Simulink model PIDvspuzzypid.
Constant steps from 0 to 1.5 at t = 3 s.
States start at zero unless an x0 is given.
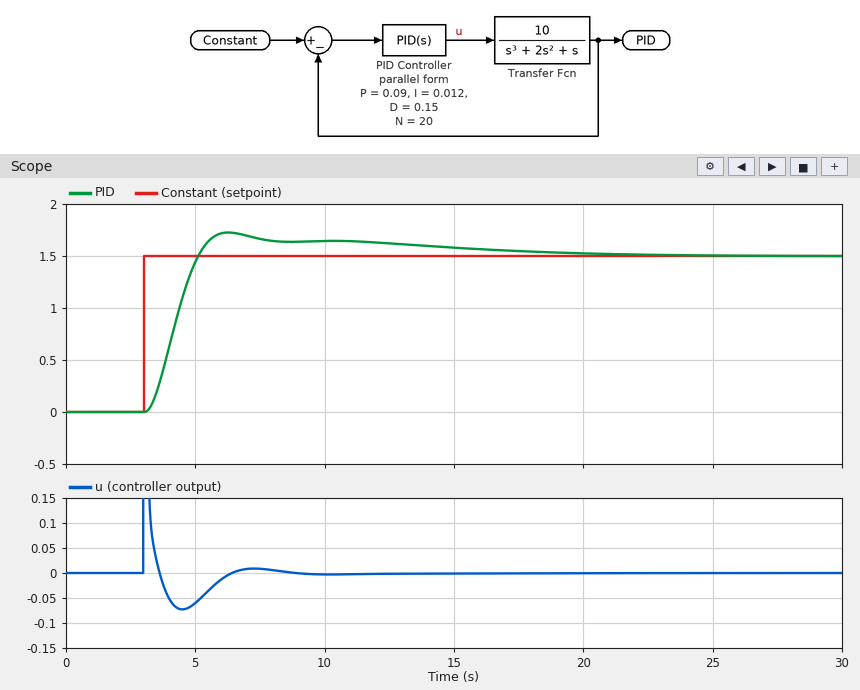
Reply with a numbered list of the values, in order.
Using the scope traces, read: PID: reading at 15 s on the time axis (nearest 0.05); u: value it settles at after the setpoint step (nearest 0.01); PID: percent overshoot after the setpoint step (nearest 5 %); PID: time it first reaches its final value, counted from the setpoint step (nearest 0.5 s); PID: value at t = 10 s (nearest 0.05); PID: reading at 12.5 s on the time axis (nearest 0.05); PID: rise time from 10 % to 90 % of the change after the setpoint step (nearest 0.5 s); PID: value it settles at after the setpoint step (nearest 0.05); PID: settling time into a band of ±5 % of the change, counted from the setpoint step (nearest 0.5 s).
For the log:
1. 1.60
2. 0.00
3. 15 %
4. 2.0 s
5. 1.65
6. 1.60
7. 1.5 s
8. 1.50
9. 12.5 s
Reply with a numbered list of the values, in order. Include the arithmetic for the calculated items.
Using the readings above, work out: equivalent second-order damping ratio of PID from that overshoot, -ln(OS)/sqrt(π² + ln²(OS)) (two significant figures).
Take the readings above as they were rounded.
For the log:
1. ln(0.15) = -1.897; 1.897 / sqrt(9.870 + 3.599) = 0.52
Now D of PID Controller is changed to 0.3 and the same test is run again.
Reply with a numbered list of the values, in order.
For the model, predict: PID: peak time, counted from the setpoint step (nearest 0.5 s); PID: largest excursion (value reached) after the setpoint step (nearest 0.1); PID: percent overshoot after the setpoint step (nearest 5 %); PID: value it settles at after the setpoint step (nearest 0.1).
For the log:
1. 2.0 s
2. 1.7
3. 10 %
4. 1.5
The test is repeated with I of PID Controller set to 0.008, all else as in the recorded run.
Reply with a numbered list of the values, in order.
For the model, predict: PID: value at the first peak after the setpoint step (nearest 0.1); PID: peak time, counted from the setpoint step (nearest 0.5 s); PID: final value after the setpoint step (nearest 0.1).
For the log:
1. 1.7
2. 3.0 s
3. 1.5
